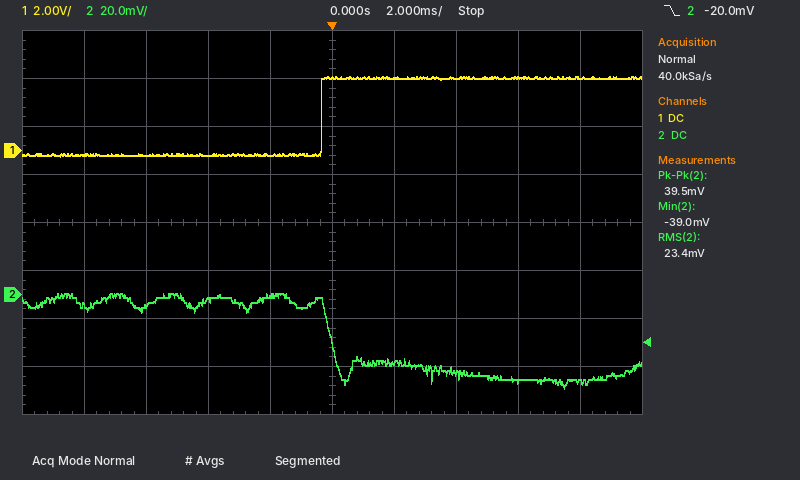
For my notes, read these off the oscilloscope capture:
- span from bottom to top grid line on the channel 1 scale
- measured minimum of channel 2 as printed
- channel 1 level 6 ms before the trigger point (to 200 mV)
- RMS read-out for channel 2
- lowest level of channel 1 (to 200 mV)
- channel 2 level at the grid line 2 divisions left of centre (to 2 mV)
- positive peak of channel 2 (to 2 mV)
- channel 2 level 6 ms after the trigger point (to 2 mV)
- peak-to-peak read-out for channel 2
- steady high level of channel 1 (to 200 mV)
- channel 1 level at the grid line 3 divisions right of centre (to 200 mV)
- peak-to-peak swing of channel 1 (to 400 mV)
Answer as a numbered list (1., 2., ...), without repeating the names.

1. 16 V
2. -39.0 mV
3. -200 mV
4. 23.4 mV
5. -200 mV
6. -2 mV
7. 0 mV
8. -36 mV
9. 39.5 mV
10. 3.0 V
11. 3.0 V
12. 3.2 V
